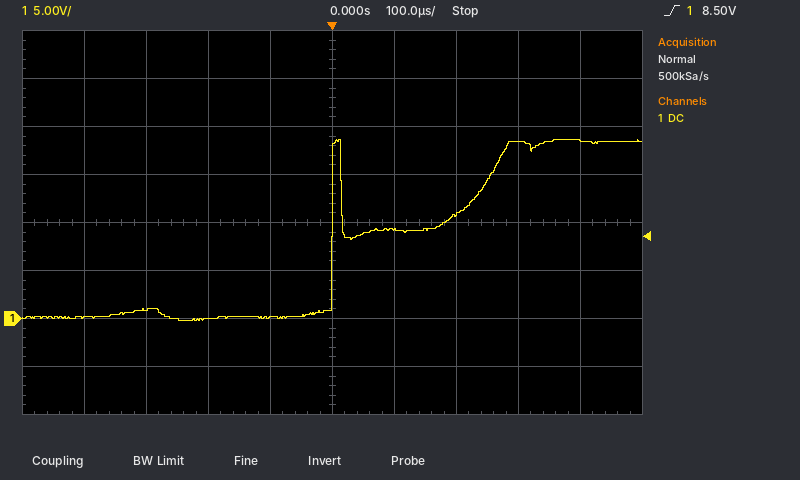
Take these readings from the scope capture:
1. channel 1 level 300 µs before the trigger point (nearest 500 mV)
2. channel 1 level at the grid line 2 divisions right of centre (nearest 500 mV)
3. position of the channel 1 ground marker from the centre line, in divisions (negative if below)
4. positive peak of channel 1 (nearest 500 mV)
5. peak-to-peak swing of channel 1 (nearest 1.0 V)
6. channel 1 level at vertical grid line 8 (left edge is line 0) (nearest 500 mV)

1.0 V
11.0 V
-2.0 div
18.5 V
19.0 V
18.5 V
